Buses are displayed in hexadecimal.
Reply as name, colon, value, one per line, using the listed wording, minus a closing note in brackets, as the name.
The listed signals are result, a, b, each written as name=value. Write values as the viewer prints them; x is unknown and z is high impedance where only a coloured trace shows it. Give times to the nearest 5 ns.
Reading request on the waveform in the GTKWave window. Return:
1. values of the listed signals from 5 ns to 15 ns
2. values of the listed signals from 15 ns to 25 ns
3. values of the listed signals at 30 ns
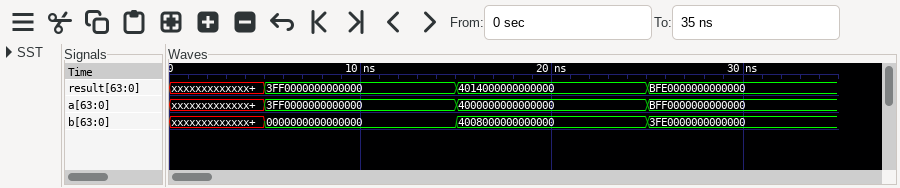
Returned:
values of the listed signals from 5 ns to 15 ns: result=3FF0000000000000, a=3FF0000000000000, b=0000000000000000
values of the listed signals from 15 ns to 25 ns: result=4014000000000000, a=4000000000000000, b=4008000000000000
values of the listed signals at 30 ns: result=BFE0000000000000, a=BFF0000000000000, b=3FE0000000000000
